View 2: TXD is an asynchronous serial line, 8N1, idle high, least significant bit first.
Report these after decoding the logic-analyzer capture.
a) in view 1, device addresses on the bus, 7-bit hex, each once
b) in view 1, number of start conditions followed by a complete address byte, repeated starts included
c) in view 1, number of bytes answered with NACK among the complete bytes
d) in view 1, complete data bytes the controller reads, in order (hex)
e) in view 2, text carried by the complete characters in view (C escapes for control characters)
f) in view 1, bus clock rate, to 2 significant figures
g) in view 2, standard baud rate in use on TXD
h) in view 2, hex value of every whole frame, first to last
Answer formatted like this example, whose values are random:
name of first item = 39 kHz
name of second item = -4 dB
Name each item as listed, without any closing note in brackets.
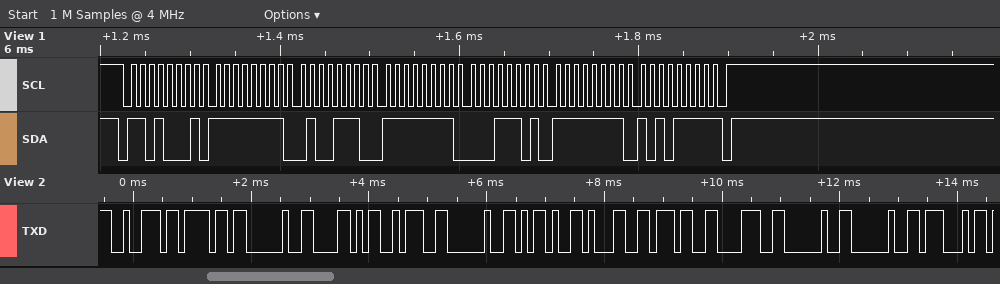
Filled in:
in view 1, device addresses on the bus, 7-bit hex, each once = 0x68
in view 1, number of start conditions followed by a complete address byte, repeated starts included = 1
in view 1, number of bytes answered with NACK among the complete bytes = 1
in view 1, complete data bytes the controller reads, in order = FF 4E FF 1D FF AF
in view 2, text carried by the complete characters in view = "ro X: -178  G"
in view 1, bus clock rate, to 2 significant figures = 100 kHz
in view 2, standard baud rate in use on TXD = 9600 baud
in view 2, hex value of every whole frame, first to last = 72 6F 20 58 3A 20 2D 31 37 38 20 20 47
